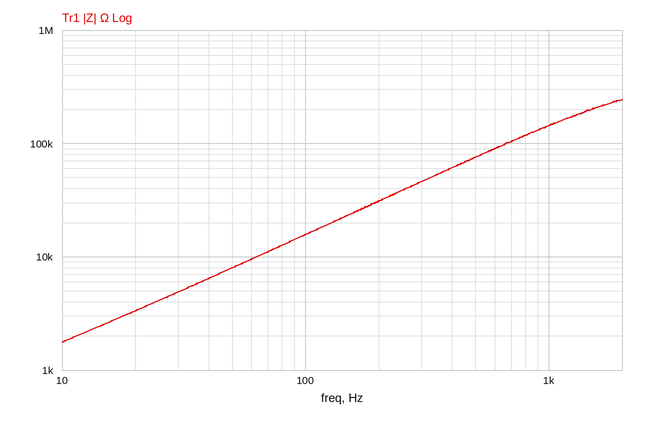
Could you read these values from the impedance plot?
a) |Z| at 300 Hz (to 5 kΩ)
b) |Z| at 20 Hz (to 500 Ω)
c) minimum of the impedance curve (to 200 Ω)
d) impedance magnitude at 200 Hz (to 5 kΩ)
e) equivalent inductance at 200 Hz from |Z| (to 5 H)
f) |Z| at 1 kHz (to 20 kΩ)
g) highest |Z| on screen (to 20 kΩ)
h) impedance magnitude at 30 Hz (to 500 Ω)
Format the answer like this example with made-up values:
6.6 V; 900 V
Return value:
45 kΩ; 3.5 kΩ; 1.8 kΩ; 30 kΩ; 25 H; 140 kΩ; 240 kΩ; 5.0 kΩ
